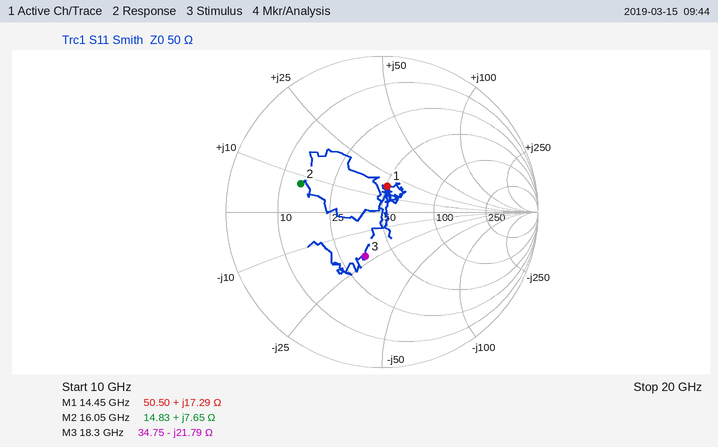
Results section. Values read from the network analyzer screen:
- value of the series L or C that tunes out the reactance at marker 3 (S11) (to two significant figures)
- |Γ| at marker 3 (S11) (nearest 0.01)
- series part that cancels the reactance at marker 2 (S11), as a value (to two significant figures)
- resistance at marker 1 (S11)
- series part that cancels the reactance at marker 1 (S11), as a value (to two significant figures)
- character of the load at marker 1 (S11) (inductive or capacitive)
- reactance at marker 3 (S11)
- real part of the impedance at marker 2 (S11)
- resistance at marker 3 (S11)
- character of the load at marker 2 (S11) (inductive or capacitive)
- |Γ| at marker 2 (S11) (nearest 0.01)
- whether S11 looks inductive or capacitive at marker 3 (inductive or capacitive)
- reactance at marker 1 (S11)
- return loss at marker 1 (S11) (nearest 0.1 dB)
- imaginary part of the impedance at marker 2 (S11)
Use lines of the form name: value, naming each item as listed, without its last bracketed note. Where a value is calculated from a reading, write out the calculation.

value of the series L or C that tunes out the reactance at marker 3 (S11): L = 21.79 Ω/(2π × 18.3 GHz) ≈ 190 pH
|Γ| at marker 3 (S11): 0.30
series part that cancels the reactance at marker 2 (S11), as a value: C = 1/(2π × 16.05 GHz × 7.65 Ω) ≈ 1.3 pF
resistance at marker 1: 50.50 Ω
series part that cancels the reactance at marker 1 (S11), as a value: C = 1/(2π × 14.45 GHz × 17.29 Ω) ≈ 637 fF, so 640 fF to two significant figures
character of the load at marker 1 (S11): inductive
reactance at marker 3: -21.79 Ω
real part of the impedance at marker 2: 14.83 Ω
resistance at marker 3: 34.75 Ω
character of the load at marker 2 (S11): inductive
|Γ| at marker 2 (S11): 0.55
whether S11 looks inductive or capacitive at marker 3: capacitive
reactance at marker 1: +17.29 Ω
return loss at marker 1 (S11): 15.4 dB
imaginary part of the impedance at marker 2: +7.65 Ω
